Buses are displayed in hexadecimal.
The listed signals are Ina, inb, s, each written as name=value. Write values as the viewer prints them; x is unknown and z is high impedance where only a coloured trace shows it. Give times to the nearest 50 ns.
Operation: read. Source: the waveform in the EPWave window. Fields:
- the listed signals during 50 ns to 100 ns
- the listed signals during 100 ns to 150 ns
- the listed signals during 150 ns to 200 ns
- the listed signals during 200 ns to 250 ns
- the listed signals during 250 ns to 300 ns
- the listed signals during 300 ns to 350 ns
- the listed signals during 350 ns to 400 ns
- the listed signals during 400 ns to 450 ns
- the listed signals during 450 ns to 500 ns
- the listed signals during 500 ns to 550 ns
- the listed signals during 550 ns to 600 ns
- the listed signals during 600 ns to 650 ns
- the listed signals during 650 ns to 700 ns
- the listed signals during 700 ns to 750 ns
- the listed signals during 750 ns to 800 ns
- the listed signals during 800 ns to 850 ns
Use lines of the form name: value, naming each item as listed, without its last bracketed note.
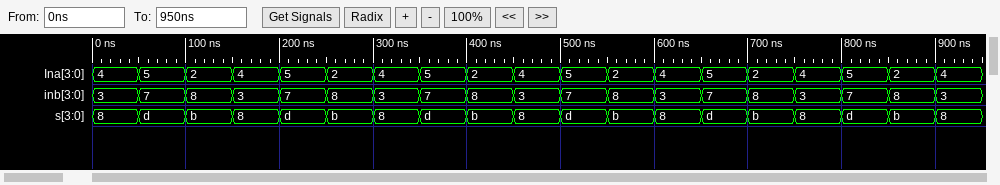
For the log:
the listed signals during 50 ns to 100 ns: Ina=5, inb=7, s=d
the listed signals during 100 ns to 150 ns: Ina=2, inb=8, s=b
the listed signals during 150 ns to 200 ns: Ina=4, inb=3, s=8
the listed signals during 200 ns to 250 ns: Ina=5, inb=7, s=d
the listed signals during 250 ns to 300 ns: Ina=2, inb=8, s=b
the listed signals during 300 ns to 350 ns: Ina=4, inb=3, s=8
the listed signals during 350 ns to 400 ns: Ina=5, inb=7, s=d
the listed signals during 400 ns to 450 ns: Ina=2, inb=8, s=b
the listed signals during 450 ns to 500 ns: Ina=4, inb=3, s=8
the listed signals during 500 ns to 550 ns: Ina=5, inb=7, s=d
the listed signals during 550 ns to 600 ns: Ina=2, inb=8, s=b
the listed signals during 600 ns to 650 ns: Ina=4, inb=3, s=8
the listed signals during 650 ns to 700 ns: Ina=5, inb=7, s=d
the listed signals during 700 ns to 750 ns: Ina=2, inb=8, s=b
the listed signals during 750 ns to 800 ns: Ina=4, inb=3, s=8
the listed signals during 800 ns to 850 ns: Ina=5, inb=7, s=d
